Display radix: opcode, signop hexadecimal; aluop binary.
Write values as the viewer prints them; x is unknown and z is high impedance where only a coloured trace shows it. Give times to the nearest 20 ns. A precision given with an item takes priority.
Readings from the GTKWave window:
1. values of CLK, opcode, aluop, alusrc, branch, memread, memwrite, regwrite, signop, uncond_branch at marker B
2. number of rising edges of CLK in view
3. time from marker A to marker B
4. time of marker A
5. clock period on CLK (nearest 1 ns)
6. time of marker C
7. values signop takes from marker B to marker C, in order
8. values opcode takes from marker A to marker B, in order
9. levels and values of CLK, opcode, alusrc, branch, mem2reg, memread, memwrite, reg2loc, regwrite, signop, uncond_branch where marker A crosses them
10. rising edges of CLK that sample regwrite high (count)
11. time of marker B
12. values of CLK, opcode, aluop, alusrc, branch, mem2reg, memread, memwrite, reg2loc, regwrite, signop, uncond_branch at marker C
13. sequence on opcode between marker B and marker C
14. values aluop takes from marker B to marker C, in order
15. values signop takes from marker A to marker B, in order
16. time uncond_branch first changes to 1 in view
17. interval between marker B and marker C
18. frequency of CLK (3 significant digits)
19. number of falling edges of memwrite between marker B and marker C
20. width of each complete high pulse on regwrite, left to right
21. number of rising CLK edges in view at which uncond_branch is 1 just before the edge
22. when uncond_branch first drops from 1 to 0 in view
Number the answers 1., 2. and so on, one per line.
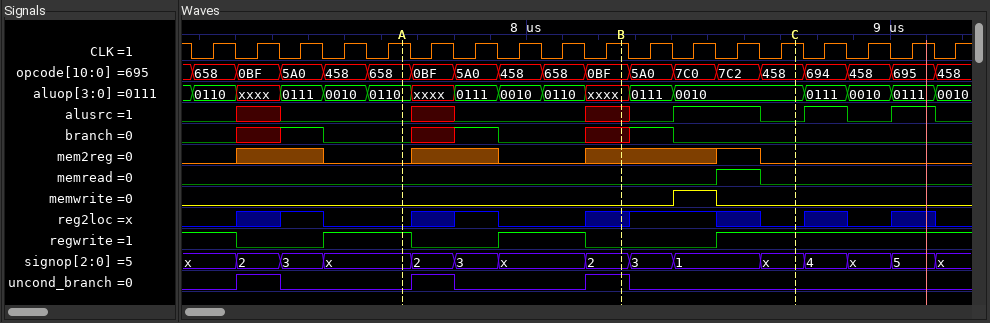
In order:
1. CLK=1, opcode=0BF, aluop=xxxx, alusrc=x, branch=x, memread=0, memwrite=0, regwrite=0, signop=2, uncond_branch=1
2. 18
3. 600 ns
4. 7660 ns
5. 120 ns
6. 8740 ns
7. 2, 3, 1, x
8. 658, 0BF, 5A0, 458, 658, 0BF
9. CLK=1, opcode=658, alusrc=0, branch=0, mem2reg=0, memread=0, memwrite=0, reg2loc=0, regwrite=1, signop=x, uncond_branch=0
10. 11
11. 8260 ns
12. CLK=1, opcode=458, aluop=0010, alusrc=0, branch=0, mem2reg=0, memread=0, memwrite=0, reg2loc=0, regwrite=1, signop=x, uncond_branch=0
13. 0BF, 5A0, 7C0, 7C2, 458
14. xxxx, 0111, 0010
15. x, 2, 3, x, 2
16. 7200 ns
17. 480 ns
18. 8.33 MHz
19. 1
20. 240 ns, 240 ns
21. 3
22. 7320 ns
